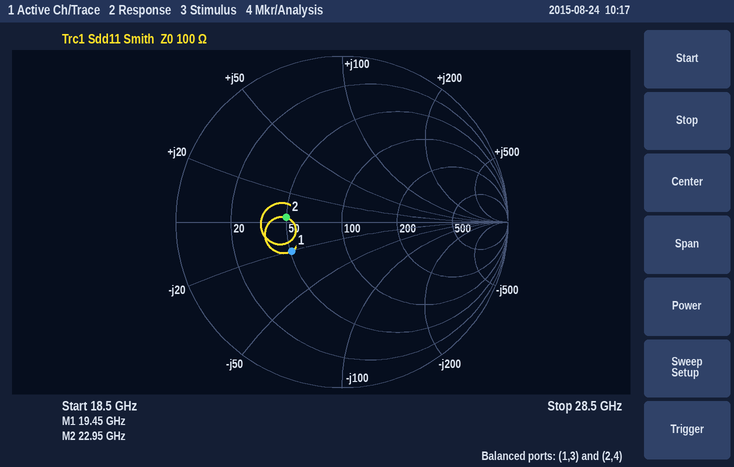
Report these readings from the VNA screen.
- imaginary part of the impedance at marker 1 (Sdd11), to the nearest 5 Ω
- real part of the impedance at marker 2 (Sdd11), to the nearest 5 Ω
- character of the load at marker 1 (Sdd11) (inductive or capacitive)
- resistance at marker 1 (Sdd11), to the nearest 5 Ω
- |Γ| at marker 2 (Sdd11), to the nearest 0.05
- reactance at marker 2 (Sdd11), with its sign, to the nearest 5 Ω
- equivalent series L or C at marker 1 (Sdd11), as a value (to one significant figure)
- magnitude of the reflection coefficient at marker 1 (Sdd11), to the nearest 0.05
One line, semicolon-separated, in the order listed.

-20 Ω; 50 Ω; capacitive; 50 Ω; 0.35; +5 Ω; 400 fF; 0.35
